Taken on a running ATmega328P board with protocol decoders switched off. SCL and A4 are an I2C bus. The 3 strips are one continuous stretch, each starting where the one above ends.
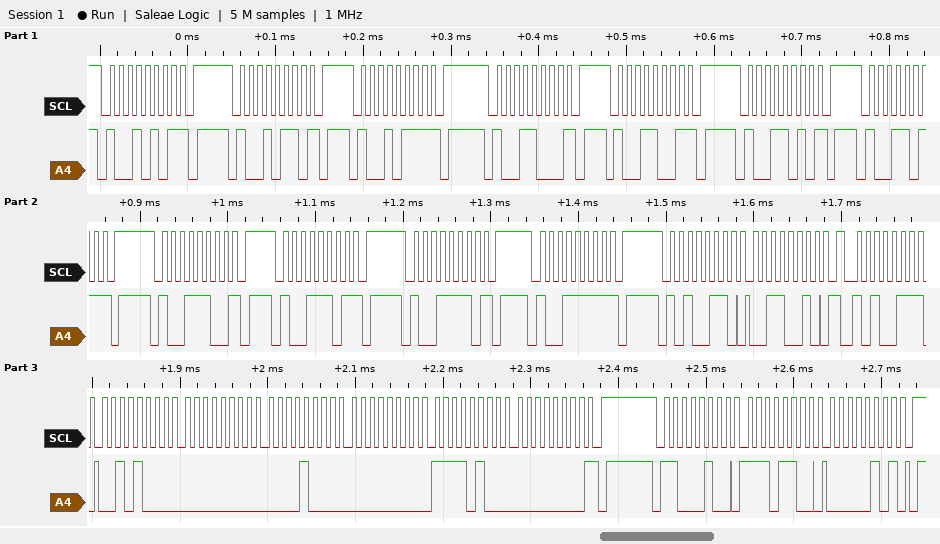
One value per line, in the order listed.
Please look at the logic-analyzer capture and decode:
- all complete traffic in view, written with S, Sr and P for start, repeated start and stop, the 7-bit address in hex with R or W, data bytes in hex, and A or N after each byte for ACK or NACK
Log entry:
S 4AR N P S 4BW N P S 4BR N P S 4CW N P S 4CR N P S 4DW N P S 4DR N P S 4EW N P S 4ER N P S 4FW N P S 4FR N P S 53W A 32 A Sr 53R A 28 A 00 A 08 A 00 A F4 A 00 N P S 62W A EC A 05 A P
